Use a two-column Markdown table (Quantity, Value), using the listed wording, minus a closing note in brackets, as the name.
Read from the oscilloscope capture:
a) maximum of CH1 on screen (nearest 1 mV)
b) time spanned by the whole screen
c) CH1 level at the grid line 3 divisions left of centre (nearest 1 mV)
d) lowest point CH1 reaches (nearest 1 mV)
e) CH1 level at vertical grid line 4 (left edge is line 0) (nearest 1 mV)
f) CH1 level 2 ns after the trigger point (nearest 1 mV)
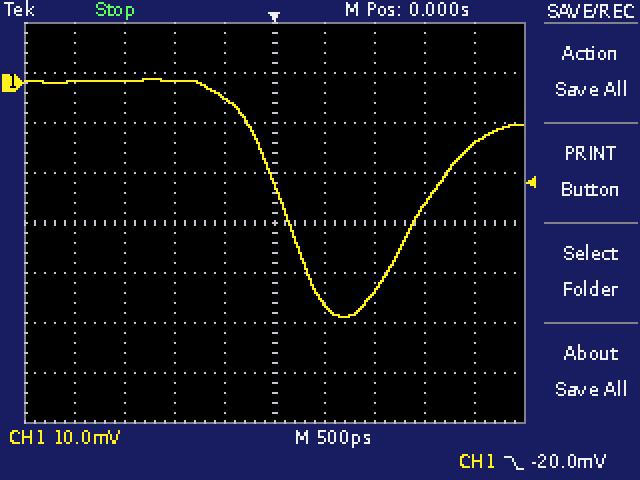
| Quantity | Value |
|---|---|
| maximum of CH1 on screen | 1 mV |
| time spanned by the whole screen | 5 ns |
| CH1 level at the grid line 3 divisions left of centre | 0 mV |
| lowest point CH1 reaches | -47 mV |
| CH1 level at vertical grid line 4 (left edge is line 0) | -3 mV |
| CH1 level 2 ns after the trigger point | -12 mV |
